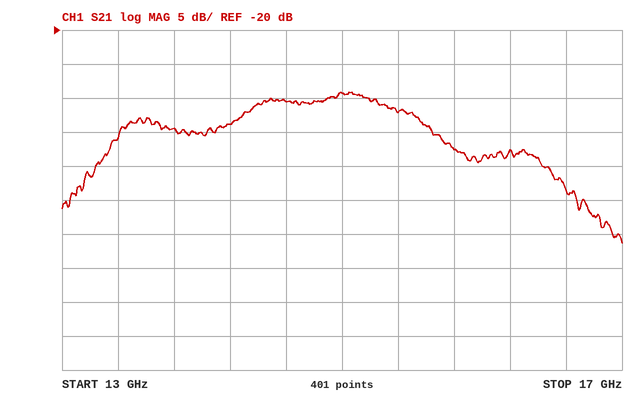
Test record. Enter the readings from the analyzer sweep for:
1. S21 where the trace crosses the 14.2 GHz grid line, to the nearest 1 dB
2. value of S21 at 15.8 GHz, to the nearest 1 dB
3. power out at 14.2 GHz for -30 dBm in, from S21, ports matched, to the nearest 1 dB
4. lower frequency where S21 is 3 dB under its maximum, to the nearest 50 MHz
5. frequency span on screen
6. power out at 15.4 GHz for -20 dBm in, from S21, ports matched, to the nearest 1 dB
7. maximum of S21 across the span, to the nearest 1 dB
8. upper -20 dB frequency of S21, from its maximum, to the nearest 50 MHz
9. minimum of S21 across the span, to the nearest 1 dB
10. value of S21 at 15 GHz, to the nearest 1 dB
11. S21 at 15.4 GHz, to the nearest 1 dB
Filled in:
-34 dB
-38 dB
-64 dBm
14.30 GHz
4 GHz
-52 dBm
-29 dB
16.90 GHz
-51 dB
-29 dB
-32 dB
